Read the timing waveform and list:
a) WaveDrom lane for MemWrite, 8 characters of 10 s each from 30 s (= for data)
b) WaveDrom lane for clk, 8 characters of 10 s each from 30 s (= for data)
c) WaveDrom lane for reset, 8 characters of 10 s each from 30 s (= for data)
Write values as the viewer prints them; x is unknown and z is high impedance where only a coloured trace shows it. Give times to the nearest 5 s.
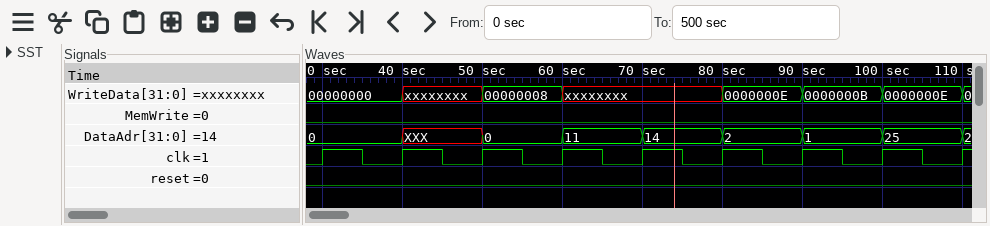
{name: 'MemWrite', wave: '0.......'}
{name: 'clk', wave: 'p.......'}
{name: 'reset', wave: '0.......'}
